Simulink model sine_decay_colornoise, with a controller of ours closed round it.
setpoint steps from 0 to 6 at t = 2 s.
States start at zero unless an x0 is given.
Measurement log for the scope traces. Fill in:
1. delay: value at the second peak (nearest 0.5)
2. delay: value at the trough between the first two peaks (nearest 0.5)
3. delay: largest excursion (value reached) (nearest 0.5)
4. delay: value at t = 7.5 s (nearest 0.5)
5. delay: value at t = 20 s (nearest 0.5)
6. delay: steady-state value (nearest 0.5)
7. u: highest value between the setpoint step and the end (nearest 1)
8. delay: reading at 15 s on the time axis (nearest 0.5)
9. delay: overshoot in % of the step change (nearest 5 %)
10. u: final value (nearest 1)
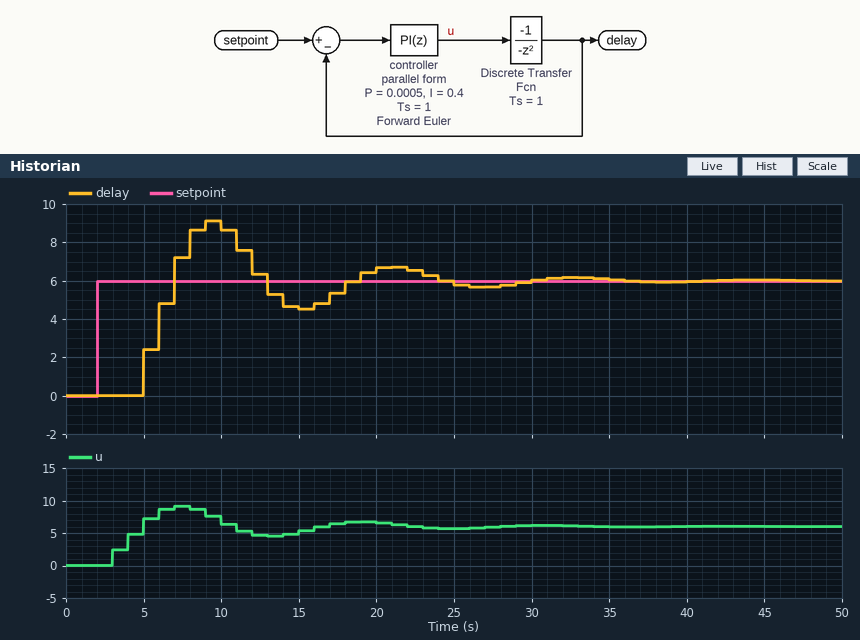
6.5
4.5
9.0
7.0
6.5
6.0
9
4.5
50 %
6
